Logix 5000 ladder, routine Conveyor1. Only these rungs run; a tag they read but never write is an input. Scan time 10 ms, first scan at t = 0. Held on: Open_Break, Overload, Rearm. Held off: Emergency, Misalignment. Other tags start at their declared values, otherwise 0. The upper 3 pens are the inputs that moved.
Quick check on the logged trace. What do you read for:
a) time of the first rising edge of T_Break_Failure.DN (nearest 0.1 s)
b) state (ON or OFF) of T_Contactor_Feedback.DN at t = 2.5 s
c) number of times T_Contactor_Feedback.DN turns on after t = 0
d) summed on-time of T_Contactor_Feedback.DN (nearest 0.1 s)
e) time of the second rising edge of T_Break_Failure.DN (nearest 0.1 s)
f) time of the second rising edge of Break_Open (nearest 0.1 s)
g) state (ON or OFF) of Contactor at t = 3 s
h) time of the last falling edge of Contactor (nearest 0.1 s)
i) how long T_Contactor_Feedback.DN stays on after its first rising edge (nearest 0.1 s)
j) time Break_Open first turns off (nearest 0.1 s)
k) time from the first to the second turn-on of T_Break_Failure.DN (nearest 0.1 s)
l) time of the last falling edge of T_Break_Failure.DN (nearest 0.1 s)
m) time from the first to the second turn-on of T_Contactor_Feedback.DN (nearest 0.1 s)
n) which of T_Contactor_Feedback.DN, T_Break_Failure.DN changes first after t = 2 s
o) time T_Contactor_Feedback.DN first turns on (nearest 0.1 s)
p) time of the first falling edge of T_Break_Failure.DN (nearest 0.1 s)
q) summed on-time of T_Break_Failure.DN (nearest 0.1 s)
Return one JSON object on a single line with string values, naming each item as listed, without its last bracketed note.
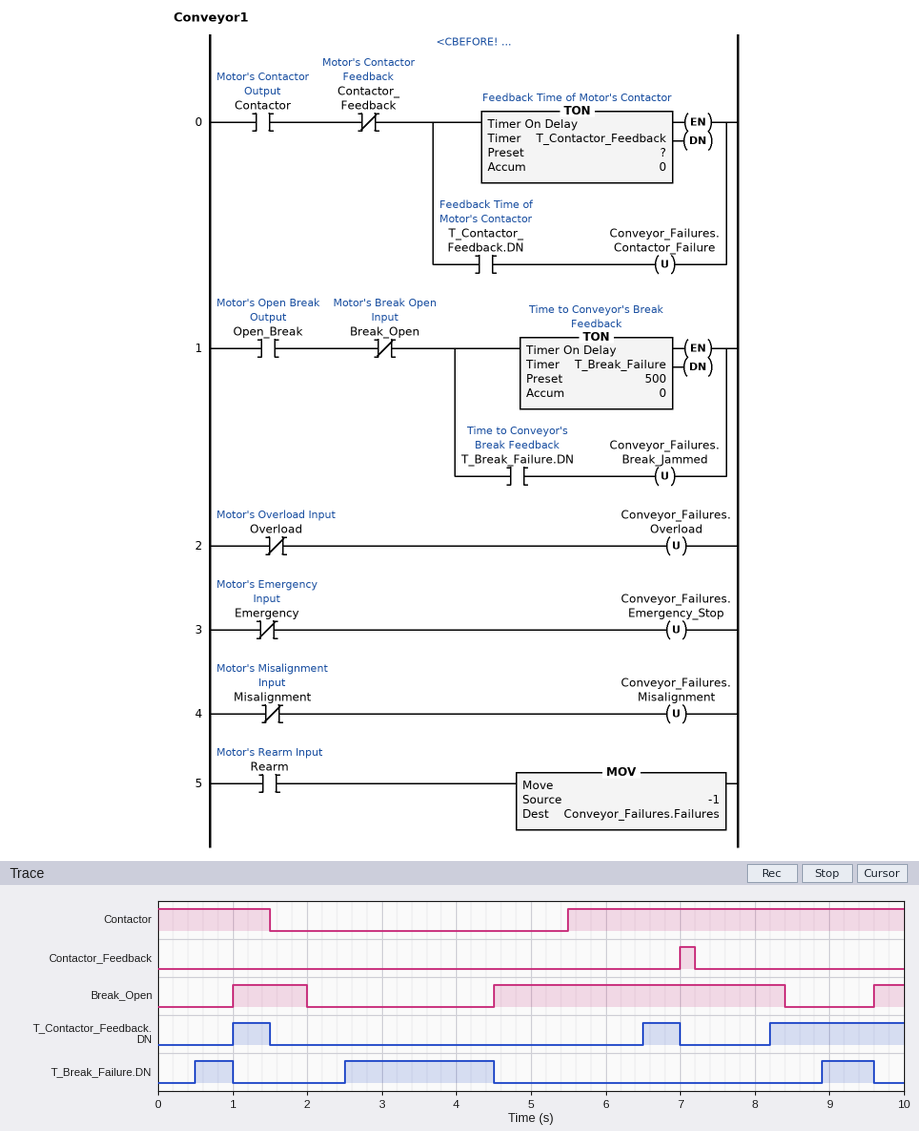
{"time of the first rising edge of T_Break_Failure.DN": "0.5 s", "state (ON or OFF) of T_Contactor_Feedback.DN at t = 2.5 s": "OFF", "number of times T_Contactor_Feedback.DN turns on after t = 0": "3", "summed on-time of T_Contactor_Feedback.DN": "2.8 s", "time of the second rising edge of T_Break_Failure.DN": "2.5 s", "time of the second rising edge of Break_Open": "4.5 s", "state (ON or OFF) of Contactor at t = 3 s": "OFF", "time of the last falling edge of Contactor": "1.5 s", "how long T_Contactor_Feedback.DN stays on after its first rising edge": "0.5 s", "time Break_Open first turns off": "2.0 s", "time from the first to the second turn-on of T_Break_Failure.DN": "2.0 s", "time of the last falling edge of T_Break_Failure.DN": "9.6 s", "time from the first to the second turn-on of T_Contactor_Feedback.DN": "5.5 s", "which of T_Contactor_Feedback.DN, T_Break_Failure.DN changes first after t = 2 s": "T_Break_Failure.DN", "time T_Contactor_Feedback.DN first turns on": "1.0 s", "time of the first falling edge of T_Break_Failure.DN": "1.0 s", "summed on-time of T_Break_Failure.DN": "3.2 s"}
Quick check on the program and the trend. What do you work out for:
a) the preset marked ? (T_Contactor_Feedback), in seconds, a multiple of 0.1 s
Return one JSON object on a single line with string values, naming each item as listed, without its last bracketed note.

{"the preset marked ? (T_Contactor_Feedback), in seconds, a multiple of 0.1 s": "1.0 s"}
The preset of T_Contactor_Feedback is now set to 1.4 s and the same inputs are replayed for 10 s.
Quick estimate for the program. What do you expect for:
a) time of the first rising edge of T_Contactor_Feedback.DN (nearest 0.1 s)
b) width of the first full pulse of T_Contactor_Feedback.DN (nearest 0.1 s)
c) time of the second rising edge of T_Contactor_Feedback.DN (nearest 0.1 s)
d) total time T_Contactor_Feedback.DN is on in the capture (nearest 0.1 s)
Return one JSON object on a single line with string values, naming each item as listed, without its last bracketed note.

{"time of the first rising edge of T_Contactor_Feedback.DN": "1.4 s", "width of the first full pulse of T_Contactor_Feedback.DN": "0.1 s", "time of the second rising edge of T_Contactor_Feedback.DN": "6.9 s", "total time T_Contactor_Feedback.DN is on in the capture": "1.6 s"}
